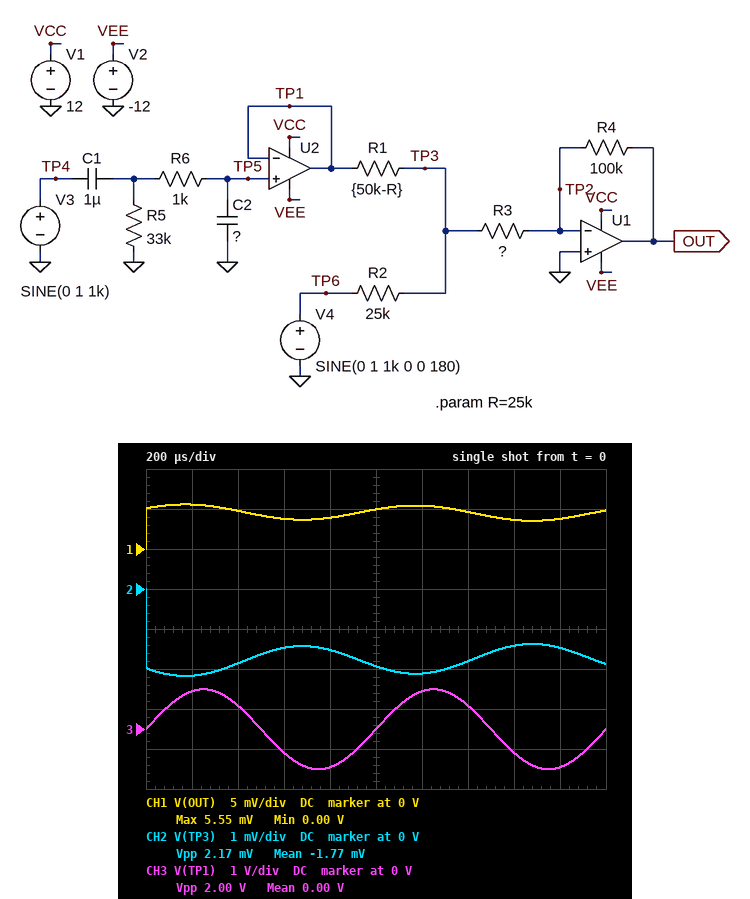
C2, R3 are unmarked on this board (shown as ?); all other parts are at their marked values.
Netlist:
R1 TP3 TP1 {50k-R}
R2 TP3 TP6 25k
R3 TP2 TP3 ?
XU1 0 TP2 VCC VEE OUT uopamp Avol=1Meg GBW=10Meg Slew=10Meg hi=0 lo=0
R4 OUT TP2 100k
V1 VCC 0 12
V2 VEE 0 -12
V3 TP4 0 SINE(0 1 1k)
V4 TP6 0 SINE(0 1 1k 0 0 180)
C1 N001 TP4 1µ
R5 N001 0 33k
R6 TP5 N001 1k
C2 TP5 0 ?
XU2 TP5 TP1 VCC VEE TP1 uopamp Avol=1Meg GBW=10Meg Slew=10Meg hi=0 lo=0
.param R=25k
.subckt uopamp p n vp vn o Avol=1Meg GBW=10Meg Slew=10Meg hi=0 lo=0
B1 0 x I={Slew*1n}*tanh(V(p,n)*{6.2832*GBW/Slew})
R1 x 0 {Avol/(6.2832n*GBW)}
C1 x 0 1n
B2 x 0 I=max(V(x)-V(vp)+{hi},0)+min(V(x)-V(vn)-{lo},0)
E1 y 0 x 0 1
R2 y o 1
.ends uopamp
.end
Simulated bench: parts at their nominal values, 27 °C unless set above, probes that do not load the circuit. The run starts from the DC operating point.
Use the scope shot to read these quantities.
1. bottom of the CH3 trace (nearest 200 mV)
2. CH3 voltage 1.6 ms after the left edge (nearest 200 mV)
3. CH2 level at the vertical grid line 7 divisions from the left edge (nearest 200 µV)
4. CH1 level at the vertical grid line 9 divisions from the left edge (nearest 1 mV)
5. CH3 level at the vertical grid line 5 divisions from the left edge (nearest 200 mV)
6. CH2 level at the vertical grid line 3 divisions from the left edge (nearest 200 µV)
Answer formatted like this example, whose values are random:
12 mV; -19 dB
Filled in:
-1.0 V; -600 mV; -1.8 mV; 4 mV; 0 V; -1.4 mV
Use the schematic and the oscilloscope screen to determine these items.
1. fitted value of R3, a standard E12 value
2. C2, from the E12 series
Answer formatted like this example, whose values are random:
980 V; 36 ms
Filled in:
39 kΩ; 820 pF
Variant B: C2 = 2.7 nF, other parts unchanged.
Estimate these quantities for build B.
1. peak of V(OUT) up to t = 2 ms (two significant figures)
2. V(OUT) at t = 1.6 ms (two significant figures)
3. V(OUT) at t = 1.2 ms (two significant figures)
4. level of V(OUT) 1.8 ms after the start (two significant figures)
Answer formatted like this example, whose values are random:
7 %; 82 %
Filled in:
17 mV; -6.8 mV; 11 mV; 5.4 mV
